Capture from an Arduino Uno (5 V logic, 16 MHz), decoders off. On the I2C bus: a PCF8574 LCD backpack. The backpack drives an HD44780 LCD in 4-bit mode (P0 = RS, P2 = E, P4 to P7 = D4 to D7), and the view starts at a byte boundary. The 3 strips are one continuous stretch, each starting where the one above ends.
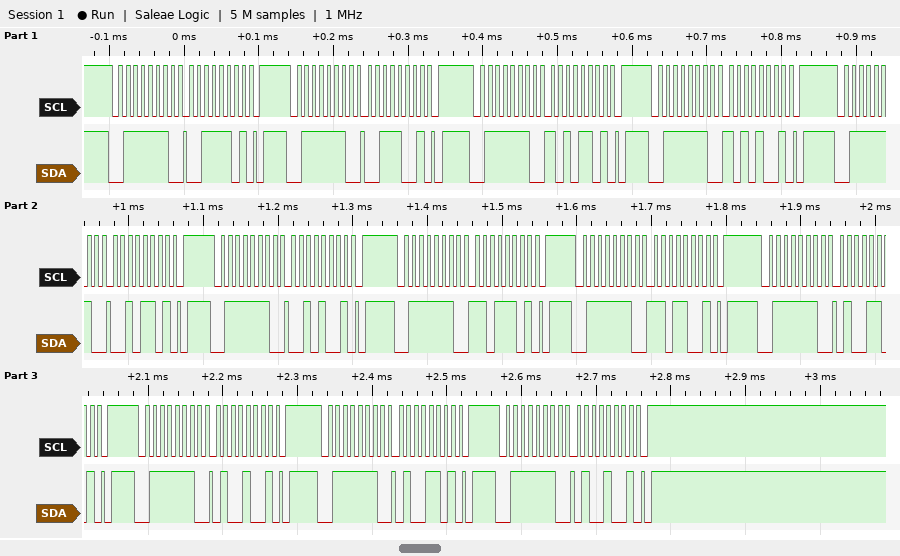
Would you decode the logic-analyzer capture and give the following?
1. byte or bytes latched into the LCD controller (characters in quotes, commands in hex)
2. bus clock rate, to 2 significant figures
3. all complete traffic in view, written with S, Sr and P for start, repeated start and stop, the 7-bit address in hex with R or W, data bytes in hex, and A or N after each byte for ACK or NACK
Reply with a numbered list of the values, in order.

1. ':' '-' 'D'
2. 100 kHz
3. S 3FW A 3D A P S 3FW A 39 A P S 3FW A AD A P S 3FW A A9 A P S 3FW A 2D A P S 3FW A 29 A P S 3FW A DD A P S 3FW A D9 A P S 3FW A 4D A P S 3FW A 49 A P S 3FW A 4D A P S 3FW A 49 A P
